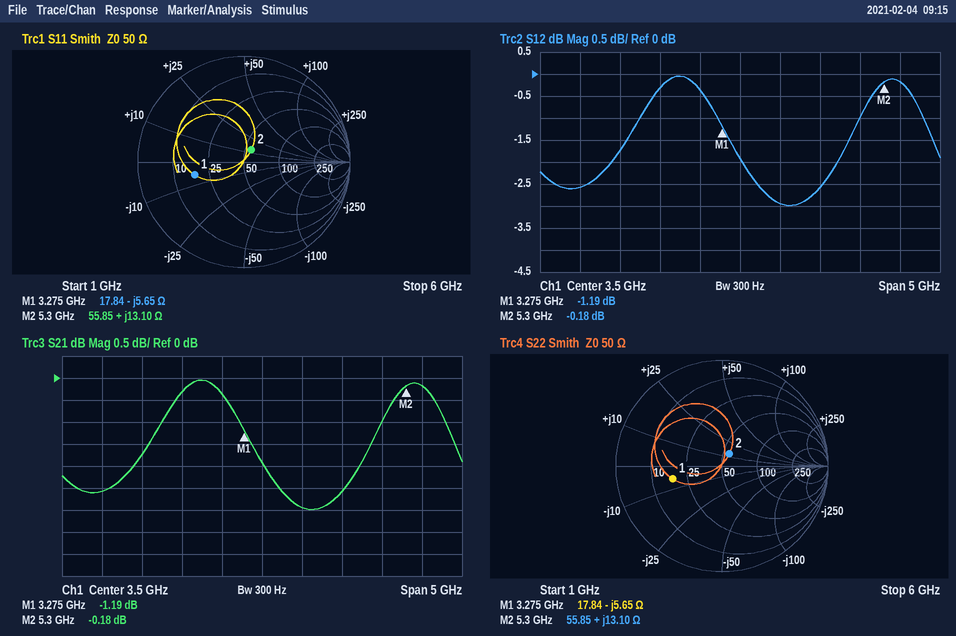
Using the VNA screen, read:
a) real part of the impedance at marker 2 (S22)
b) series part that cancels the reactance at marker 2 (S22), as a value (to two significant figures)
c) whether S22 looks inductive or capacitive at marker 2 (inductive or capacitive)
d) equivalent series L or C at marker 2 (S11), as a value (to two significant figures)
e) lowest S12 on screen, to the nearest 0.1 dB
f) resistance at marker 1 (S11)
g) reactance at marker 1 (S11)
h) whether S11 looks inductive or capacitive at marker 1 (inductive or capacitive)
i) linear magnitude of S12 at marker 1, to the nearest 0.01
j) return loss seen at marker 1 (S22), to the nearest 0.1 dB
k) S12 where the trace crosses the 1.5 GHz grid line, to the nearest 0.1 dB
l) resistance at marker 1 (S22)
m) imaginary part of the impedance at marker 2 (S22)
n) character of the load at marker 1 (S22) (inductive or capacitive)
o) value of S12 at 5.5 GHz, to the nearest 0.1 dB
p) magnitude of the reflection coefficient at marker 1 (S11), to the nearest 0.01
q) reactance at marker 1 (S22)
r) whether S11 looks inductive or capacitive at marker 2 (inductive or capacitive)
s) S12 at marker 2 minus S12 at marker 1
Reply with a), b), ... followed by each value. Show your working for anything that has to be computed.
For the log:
a) 55.85 Ω
b) C = 1/(2π × 5.3 GHz × 13.1 Ω) ≈ 2.3 pF
c) inductive
d) L = 13.1 Ω/(2π × 5.3 GHz) ≈ 393 pH, so 390 pH to two significant figures
e) -3.0 dB
f) 17.84 Ω
g) -5.65 Ω
h) capacitive
i) 10^(-1.19/20) ≈ 0.87
j) 6.4 dB
k) -2.6 dB
l) 17.84 Ω
m) +13.10 Ω
n) capacitive
o) -0.2 dB
p) 0.48
q) -5.65 Ω
r) inductive
s) -0.18 − (-1.19) = 1.01 dB
